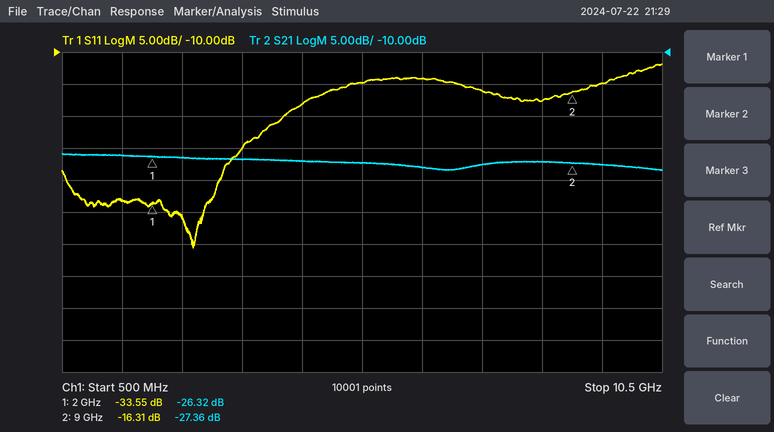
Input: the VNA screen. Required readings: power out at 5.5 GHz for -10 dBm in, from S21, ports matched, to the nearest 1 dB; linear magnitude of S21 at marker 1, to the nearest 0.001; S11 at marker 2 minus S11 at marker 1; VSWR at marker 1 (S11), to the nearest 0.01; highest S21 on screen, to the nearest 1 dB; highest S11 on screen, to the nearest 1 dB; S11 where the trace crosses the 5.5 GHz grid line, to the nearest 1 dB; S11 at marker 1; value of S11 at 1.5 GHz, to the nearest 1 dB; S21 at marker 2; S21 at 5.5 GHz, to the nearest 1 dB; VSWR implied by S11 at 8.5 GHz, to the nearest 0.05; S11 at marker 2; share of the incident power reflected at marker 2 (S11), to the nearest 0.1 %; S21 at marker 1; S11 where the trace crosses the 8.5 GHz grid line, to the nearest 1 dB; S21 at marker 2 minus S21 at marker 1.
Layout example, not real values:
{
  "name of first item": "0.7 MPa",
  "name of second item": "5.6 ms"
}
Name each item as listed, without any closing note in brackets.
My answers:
{
  "power out at 5.5 GHz for -10 dBm in, from S21, ports matched, to the nearest 1 dB": "-37 dBm",
  "linear magnitude of S21 at marker 1, to the nearest 0.001": "0.048",
  "S11 at marker 2 minus S11 at marker 1": "17.24 dB",
  "VSWR at marker 1 (S11), to the nearest 0.01": "1.04",
  "highest S21 on screen, to the nearest 1 dB": "-26 dB",
  "highest S11 on screen, to the nearest 1 dB": "-12 dB",
  "S11 where the trace crosses the 5.5 GHz grid line, to the nearest 1 dB": "-15 dB",
  "S11 at marker 1": "-33.55 dB",
  "value of S11 at 1.5 GHz, to the nearest 1 dB": "-33 dB",
  "S21 at marker 2": "-27.36 dB",
  "S21 at 5.5 GHz, to the nearest 1 dB": "-27 dB",
  "VSWR implied by S11 at 8.5 GHz, to the nearest 0.05": "1.30",
  "S11 at marker 2": "-16.31 dB",
  "share of the incident power reflected at marker 2 (S11), to the nearest 0.1 %": "2.3 %",
  "S21 at marker 1": "-26.32 dB",
  "S11 where the trace crosses the 8.5 GHz grid line, to the nearest 1 dB": "-18 dB",
  "S21 at marker 2 minus S21 at marker 1": "-1.04 dB"
}
